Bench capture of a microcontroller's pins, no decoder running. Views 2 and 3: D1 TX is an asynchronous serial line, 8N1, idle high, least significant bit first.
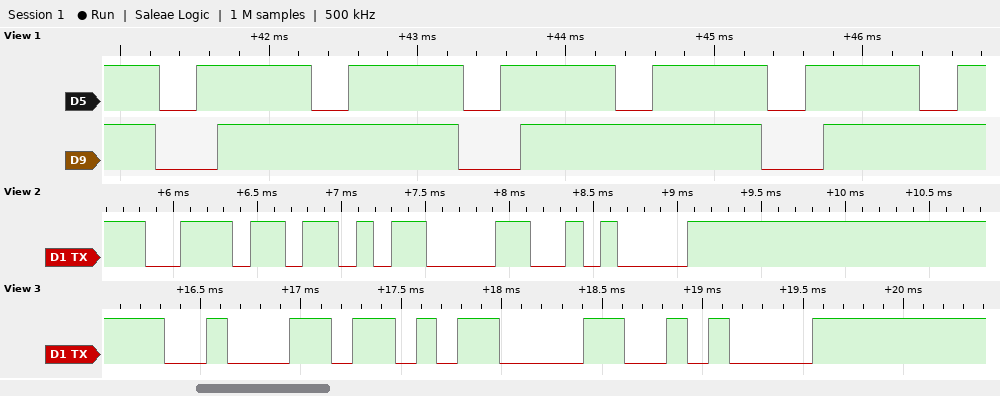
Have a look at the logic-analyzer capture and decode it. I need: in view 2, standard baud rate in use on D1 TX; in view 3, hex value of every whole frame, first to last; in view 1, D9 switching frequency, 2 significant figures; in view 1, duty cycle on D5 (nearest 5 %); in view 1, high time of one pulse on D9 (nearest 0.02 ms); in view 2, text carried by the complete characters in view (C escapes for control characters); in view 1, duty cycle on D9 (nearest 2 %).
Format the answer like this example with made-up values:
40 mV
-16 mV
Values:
9600 baud
62 0D 0A
490 Hz
75 %
1.62 ms
"n\r\n"
80 %
